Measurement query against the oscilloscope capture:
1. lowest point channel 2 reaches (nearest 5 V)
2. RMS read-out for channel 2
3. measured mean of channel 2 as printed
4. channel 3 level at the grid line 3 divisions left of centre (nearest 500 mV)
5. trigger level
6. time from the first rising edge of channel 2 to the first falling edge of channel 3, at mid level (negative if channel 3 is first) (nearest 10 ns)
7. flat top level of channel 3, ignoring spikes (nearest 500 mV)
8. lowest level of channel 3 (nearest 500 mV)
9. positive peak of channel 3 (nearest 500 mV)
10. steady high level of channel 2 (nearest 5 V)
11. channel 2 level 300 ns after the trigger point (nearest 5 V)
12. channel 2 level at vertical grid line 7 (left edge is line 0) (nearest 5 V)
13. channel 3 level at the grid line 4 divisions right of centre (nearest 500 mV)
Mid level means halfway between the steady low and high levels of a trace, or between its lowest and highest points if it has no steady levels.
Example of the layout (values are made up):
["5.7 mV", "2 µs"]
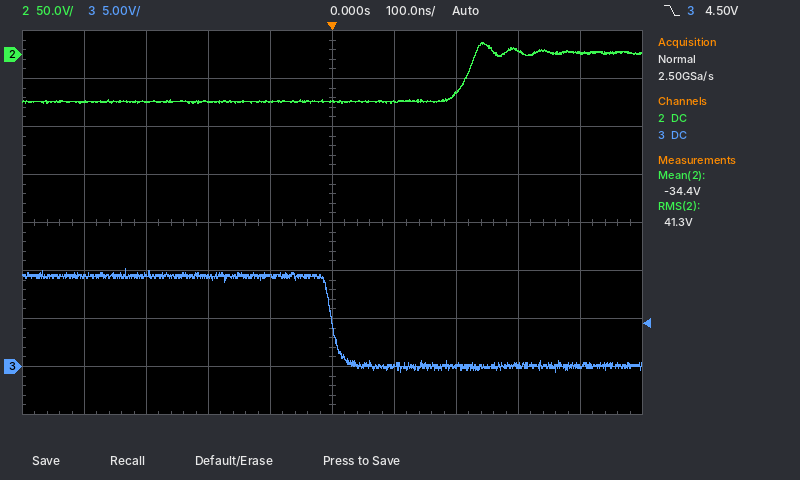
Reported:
["-50 V", "41.3 V", "-34.4 V", "9.5 V", "4.50 V", "-220 ns", "9.5 V", "-500 mV", "10.0 V", "0 V", "5 V", "-40 V", "0.0 V"]
